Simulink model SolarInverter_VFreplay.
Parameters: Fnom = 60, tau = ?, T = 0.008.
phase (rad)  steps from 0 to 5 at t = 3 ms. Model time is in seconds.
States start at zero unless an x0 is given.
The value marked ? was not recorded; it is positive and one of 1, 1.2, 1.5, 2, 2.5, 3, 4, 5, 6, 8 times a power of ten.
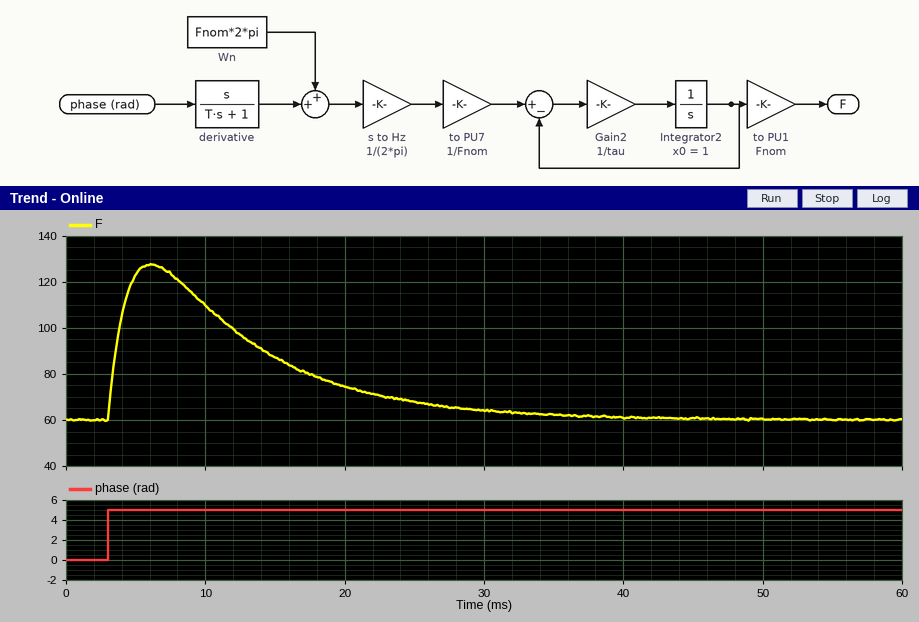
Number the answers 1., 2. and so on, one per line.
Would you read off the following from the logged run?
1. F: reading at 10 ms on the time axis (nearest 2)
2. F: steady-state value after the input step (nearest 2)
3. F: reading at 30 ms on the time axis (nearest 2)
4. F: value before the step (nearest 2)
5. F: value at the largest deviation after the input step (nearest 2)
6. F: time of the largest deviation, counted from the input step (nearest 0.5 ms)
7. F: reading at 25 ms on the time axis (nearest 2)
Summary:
1. 110
2. 60
3. 64
4. 60
5. 128
6. 3.0 ms
7. 68
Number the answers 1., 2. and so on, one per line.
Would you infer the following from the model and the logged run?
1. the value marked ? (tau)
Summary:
1. 0.0015
